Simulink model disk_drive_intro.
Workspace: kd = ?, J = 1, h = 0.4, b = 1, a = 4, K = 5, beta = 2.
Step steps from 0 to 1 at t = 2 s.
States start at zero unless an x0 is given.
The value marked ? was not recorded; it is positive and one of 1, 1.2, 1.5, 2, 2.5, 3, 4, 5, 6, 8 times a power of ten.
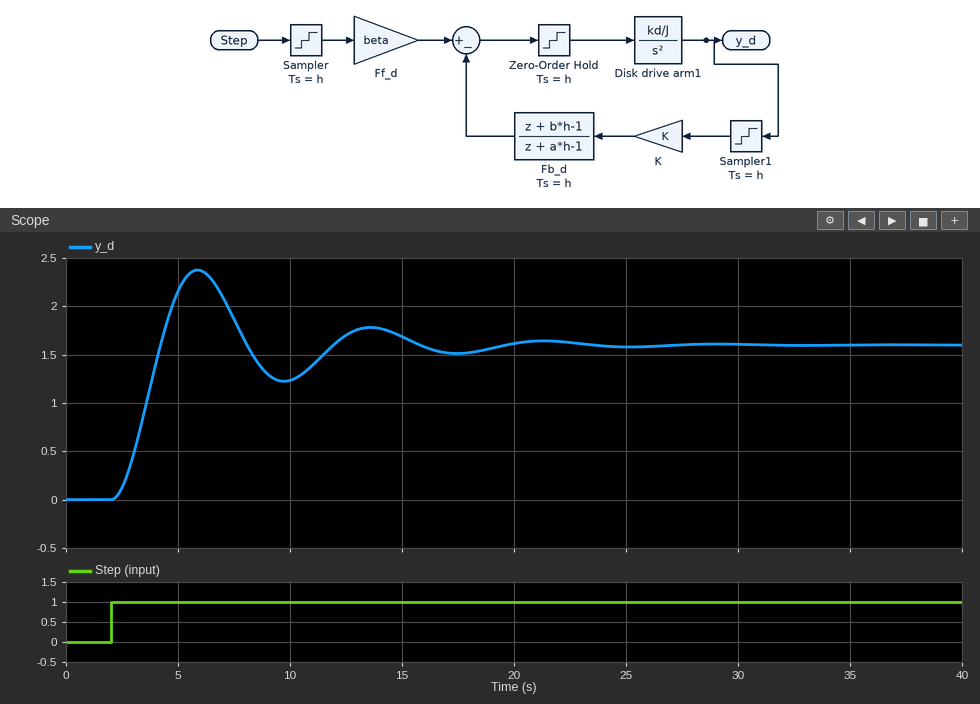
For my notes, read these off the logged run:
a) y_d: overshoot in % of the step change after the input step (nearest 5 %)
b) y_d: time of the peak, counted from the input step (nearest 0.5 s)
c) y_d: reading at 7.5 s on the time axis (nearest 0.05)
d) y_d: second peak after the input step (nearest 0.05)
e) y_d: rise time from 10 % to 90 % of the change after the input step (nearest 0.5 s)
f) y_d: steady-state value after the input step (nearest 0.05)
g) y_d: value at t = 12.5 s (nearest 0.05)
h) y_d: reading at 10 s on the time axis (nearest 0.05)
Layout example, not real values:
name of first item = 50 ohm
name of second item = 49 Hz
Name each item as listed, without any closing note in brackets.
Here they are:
y_d: overshoot in % of the step change after the input step = 50 %
y_d: time of the peak, counted from the input step = 4.0 s
y_d: reading at 7.5 s on the time axis = 1.85
y_d: second peak after the input step = 1.80
y_d: rise time from 10 % to 90 % of the change after the input step = 1.5 s
y_d: steady-state value after the input step = 1.60
y_d: value at t = 12.5 s = 1.70
y_d: reading at 10 s on the time axis = 1.25
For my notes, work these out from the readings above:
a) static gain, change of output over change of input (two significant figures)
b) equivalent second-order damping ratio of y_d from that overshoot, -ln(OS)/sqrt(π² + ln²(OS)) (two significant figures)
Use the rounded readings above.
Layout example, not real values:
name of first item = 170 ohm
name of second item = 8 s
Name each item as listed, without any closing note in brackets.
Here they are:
static gain, change of output over change of input = 1.6
equivalent second-order damping ratio of y_d from that overshoot, -ln(OS)/sqrt(π² + ln²(OS)) = 0.22
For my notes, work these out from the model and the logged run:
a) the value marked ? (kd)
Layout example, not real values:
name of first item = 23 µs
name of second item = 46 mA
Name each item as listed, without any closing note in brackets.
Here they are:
the value marked ? = 0.5
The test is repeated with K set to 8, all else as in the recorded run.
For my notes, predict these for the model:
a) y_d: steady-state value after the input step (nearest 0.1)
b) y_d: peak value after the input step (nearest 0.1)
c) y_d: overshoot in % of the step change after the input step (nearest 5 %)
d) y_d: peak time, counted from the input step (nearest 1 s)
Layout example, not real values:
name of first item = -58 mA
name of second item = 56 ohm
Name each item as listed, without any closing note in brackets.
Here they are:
y_d: steady-state value after the input step = 1.0
y_d: peak value after the input step = 1.4
y_d: overshoot in % of the step change after the input step = 40 %
y_d: peak time, counted from the input step = 3 s
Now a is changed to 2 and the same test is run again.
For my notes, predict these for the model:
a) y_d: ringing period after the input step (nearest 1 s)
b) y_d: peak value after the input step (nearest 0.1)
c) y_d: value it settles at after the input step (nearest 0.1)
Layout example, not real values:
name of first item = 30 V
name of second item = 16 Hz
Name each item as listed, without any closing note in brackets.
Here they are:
y_d: ringing period after the input step = 5 s
y_d: peak value after the input step = 1.3
y_d: value it settles at after the input step = 0.8
